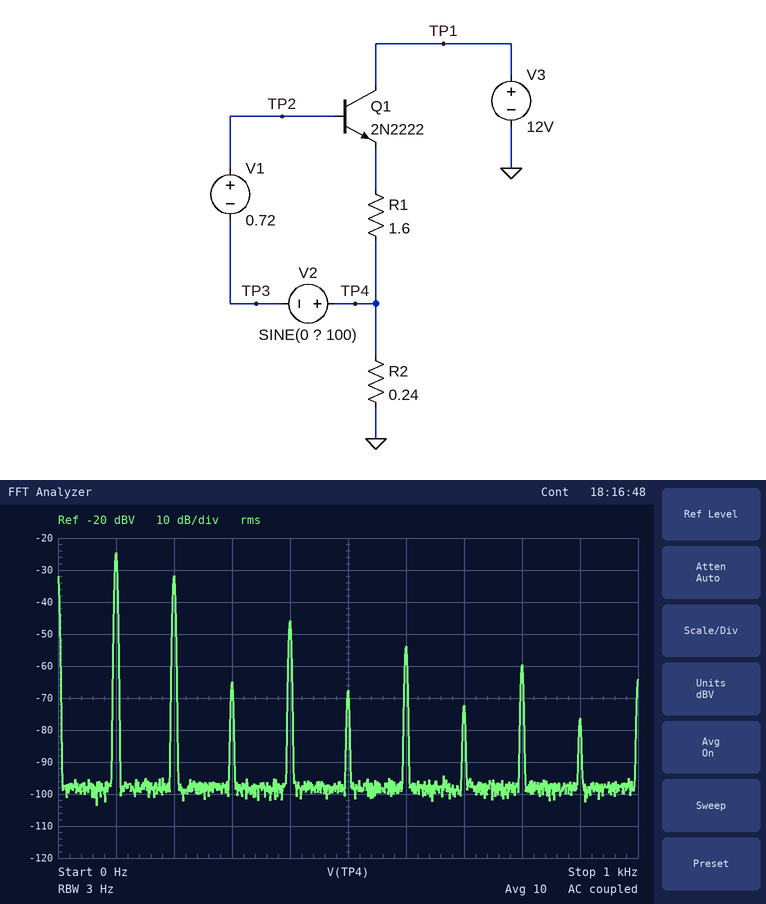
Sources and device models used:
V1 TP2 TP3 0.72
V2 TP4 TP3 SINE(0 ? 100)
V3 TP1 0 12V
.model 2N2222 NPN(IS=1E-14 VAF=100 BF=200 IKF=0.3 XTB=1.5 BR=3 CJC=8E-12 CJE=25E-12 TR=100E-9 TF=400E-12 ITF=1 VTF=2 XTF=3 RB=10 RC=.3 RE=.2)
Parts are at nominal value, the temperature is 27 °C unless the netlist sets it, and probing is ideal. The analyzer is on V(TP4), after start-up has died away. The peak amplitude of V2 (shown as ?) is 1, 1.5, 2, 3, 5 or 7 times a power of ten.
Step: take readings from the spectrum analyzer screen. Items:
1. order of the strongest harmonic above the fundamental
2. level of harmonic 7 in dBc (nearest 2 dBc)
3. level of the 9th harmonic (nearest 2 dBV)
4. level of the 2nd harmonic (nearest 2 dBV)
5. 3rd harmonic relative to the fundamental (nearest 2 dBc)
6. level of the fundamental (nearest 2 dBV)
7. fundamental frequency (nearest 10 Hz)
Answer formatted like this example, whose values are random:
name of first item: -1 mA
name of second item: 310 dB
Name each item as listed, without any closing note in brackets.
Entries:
order of the strongest harmonic above the fundamental: 2
level of harmonic 7 in dBc: -48 dBc
level of the 9th harmonic: -76 dBV
level of the 2nd harmonic: -32 dBV
3rd harmonic relative to the fundamental: -40 dBc
level of the fundamental: -24 dBV
fundamental frequency: 100 Hz
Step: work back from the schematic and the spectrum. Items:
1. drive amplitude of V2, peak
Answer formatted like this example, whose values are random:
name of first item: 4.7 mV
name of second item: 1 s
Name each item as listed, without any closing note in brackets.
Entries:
drive amplitude of V2, peak: 1.5 V
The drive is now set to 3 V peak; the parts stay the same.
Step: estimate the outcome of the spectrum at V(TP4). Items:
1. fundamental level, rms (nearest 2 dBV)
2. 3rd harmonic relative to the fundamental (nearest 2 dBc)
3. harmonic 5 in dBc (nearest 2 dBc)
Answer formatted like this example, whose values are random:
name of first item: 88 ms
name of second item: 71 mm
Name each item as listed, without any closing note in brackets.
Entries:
fundamental level, rms: -18 dBV
3rd harmonic relative to the fundamental: -44 dBc
harmonic 5 in dBc: -50 dBc
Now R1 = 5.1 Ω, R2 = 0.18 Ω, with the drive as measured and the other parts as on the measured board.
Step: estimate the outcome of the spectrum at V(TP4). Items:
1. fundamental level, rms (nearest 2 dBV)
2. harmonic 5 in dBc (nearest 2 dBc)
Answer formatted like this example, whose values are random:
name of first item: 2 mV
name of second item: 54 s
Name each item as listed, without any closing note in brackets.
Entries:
fundamental level, rms: -36 dBV
harmonic 5 in dBc: -50 dBc
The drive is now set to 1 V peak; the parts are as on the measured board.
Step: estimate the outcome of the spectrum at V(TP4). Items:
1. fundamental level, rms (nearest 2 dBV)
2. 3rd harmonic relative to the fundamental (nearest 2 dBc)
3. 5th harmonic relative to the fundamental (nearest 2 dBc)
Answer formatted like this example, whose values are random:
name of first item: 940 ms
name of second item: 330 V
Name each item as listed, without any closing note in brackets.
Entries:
fundamental level, rms: -28 dBV
3rd harmonic relative to the fundamental: -36 dBc
5th harmonic relative to the fundamental: -42 dBc
